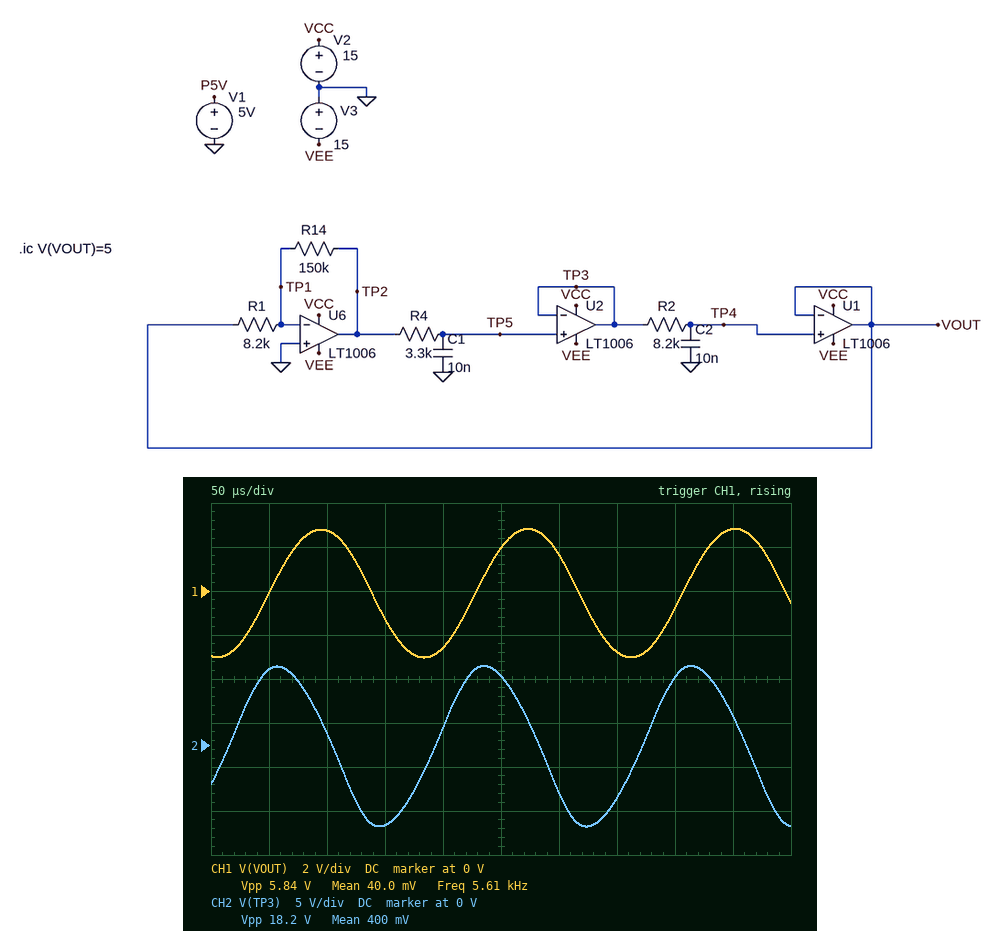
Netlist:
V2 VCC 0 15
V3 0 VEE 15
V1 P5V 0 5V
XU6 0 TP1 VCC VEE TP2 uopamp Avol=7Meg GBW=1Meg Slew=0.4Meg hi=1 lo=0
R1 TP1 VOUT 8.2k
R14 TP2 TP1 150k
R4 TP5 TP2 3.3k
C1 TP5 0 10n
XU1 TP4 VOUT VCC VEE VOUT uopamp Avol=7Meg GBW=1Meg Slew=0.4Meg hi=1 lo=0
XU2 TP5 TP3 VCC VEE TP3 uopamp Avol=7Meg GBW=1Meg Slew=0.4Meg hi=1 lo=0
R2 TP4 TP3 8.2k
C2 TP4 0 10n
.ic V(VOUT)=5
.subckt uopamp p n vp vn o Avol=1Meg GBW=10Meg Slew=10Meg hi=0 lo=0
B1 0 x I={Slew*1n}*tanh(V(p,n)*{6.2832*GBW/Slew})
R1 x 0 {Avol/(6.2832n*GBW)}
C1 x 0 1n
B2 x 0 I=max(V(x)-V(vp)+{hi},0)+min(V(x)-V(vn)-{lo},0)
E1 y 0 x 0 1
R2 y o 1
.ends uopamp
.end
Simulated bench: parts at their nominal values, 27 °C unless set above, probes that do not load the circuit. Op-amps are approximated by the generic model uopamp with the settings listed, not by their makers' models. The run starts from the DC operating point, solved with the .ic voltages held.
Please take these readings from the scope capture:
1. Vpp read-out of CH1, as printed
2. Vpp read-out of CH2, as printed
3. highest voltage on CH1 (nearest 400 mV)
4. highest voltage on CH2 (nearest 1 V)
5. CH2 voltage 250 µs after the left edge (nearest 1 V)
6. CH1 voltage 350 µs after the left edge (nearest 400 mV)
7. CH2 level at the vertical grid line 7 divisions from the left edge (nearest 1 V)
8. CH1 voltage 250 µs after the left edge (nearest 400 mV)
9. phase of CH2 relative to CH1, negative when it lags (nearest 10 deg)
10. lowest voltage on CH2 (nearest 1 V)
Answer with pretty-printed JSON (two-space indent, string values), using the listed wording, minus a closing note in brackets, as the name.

{
  "Vpp read-out of CH1, as printed": "5.84 V",
  "Vpp read-out of CH2, as printed": "18.2 V",
  "highest voltage on CH1": "2.8 V",
  "highest voltage on CH2": "9 V",
  "CH2 voltage 250 µs after the left edge": "8 V",
  "CH1 voltage 350 µs after the left edge": "-2.8 V",
  "CH2 level at the vertical grid line 7 divisions from the left edge": "-6 V",
  "CH1 voltage 250 µs after the left edge": "2.0 V",
  "phase of CH2 relative to CH1, negative when it lags": "70 deg",
  "lowest voltage on CH2": "-9 V"
}
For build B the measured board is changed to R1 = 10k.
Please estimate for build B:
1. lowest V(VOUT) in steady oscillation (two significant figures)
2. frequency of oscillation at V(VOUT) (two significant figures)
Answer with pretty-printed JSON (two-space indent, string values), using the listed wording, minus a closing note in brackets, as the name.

{
  "lowest V(VOUT) in steady oscillation": "-2.7 V",
  "frequency of oscillation at V(VOUT)": "5.9 kHz"
}
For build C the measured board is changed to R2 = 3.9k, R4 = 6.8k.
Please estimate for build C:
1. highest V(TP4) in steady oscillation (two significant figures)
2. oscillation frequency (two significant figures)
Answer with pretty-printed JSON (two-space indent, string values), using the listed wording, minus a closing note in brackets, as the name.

{
  "highest V(TP4) in steady oscillation": "3.1 V",
  "oscillation frequency": "5.5 kHz"
}
